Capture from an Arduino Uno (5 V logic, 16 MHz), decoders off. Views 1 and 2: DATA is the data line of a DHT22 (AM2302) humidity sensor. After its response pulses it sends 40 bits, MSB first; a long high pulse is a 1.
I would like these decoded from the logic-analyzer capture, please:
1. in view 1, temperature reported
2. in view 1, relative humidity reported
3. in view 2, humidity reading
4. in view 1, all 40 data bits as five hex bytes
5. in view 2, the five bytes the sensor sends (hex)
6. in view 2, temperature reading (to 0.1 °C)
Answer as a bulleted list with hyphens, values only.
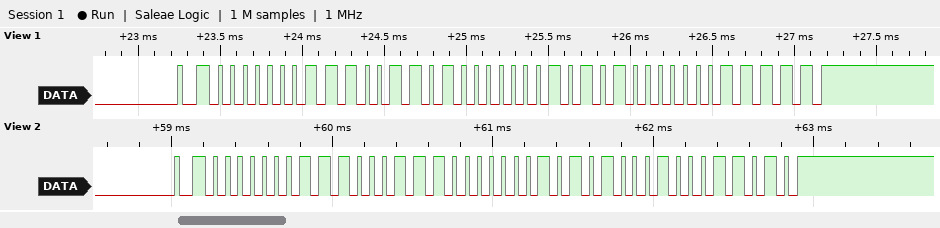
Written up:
- 33.6 °C
- 46.1 %
- 45.5 %
- 01 CD 01 50 1F
- 01 C7 01 51 1A
- 33.7 °C
